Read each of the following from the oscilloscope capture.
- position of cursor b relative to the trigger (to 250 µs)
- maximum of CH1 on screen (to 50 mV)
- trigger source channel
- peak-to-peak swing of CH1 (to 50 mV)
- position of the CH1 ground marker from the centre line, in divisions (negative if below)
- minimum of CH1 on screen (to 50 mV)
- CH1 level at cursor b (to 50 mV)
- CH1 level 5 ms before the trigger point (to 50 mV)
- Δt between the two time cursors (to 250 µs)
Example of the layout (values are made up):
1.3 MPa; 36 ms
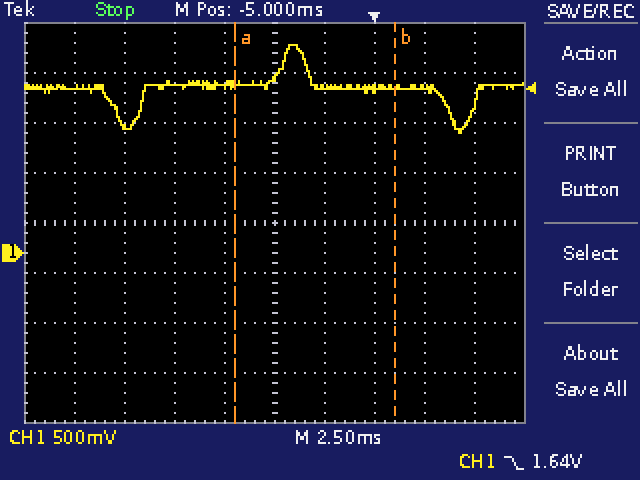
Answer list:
+1.00 ms; 2.10 V; CH1; 900 mV; -0.6 div; 1.20 V; 1.65 V; 1.75 V; 8.00 ms
